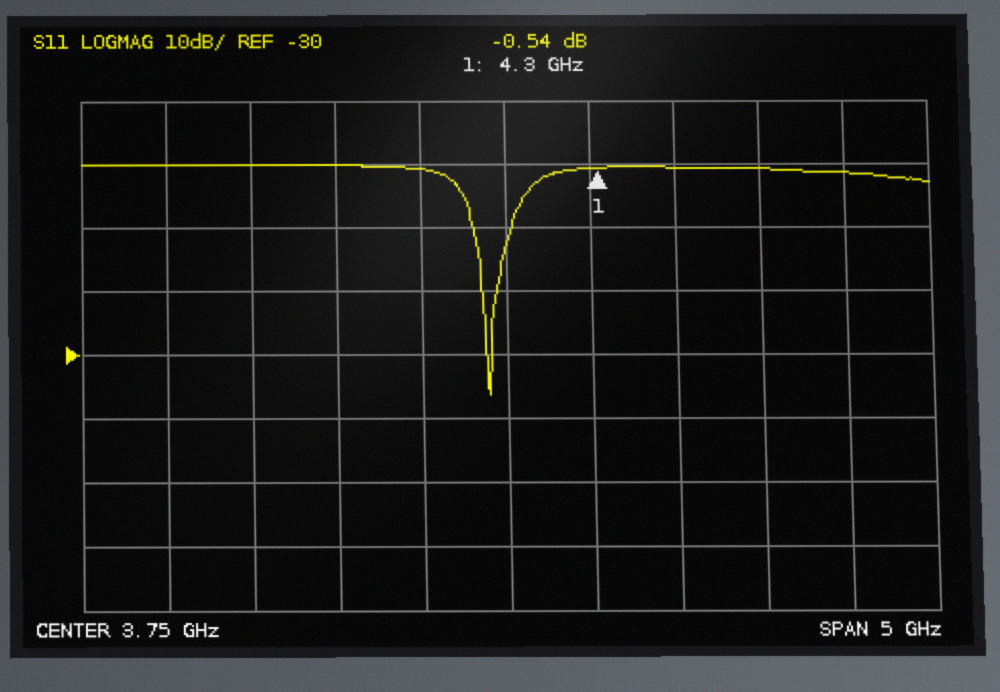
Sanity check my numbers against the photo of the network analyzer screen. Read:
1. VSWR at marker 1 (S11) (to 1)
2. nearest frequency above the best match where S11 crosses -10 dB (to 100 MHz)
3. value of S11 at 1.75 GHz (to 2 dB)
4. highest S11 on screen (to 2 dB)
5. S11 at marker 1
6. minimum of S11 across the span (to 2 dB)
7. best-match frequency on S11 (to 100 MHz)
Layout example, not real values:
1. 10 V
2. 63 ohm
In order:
1. 32
2. 3.8 GHz
3. 0 dB
4. 0 dB
5. -0.54 dB
6. -36 dB
7. 3.6 GHz
